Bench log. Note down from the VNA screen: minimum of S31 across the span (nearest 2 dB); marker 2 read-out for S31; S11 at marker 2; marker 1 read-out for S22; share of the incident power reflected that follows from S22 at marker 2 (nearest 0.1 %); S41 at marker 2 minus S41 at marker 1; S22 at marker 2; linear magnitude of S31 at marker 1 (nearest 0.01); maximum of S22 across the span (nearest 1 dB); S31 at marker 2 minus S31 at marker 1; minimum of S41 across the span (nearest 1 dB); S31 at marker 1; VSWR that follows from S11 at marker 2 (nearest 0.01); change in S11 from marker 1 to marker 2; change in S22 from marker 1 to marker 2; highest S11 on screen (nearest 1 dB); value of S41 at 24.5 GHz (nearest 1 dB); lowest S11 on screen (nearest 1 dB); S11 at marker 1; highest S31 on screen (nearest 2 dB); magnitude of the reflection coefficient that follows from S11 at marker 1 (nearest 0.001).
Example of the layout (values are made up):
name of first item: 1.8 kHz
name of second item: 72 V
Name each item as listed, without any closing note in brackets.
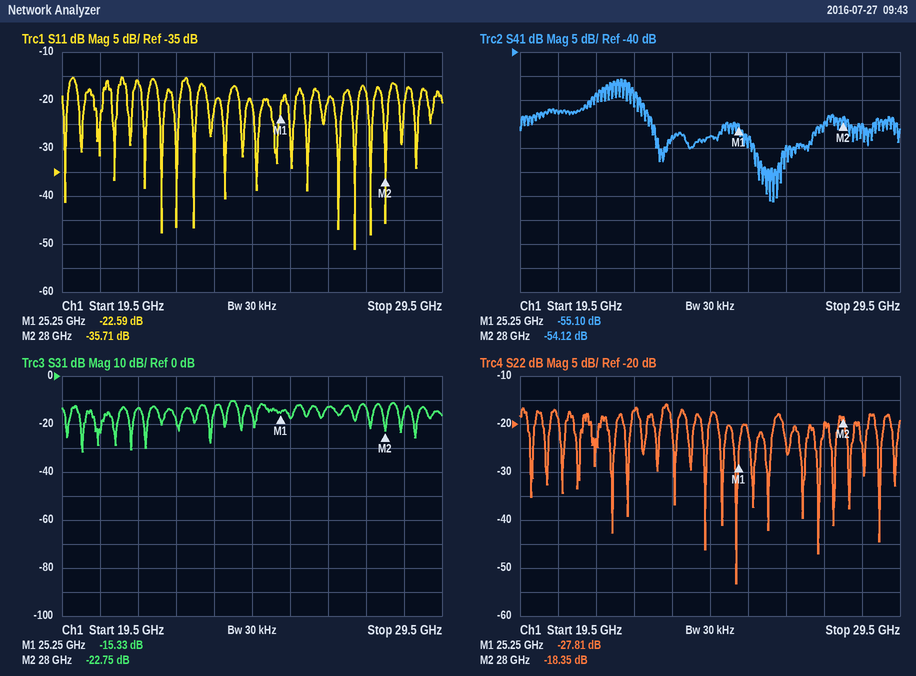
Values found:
minimum of S31 across the span: -32 dB
marker 2 read-out for S31: -22.75 dB
S11 at marker 2: -35.71 dB
marker 1 read-out for S22: -27.81 dB
share of the incident power reflected that follows from S22 at marker 2: 1.5 %
S41 at marker 2 minus S41 at marker 1: 0.98 dB
S22 at marker 2: -18.35 dB
linear magnitude of S31 at marker 1: 0.17
maximum of S22 across the span: -16 dB
S31 at marker 2 minus S31 at marker 1: -7.42 dB
minimum of S41 across the span: -71 dB
S31 at marker 1: -15.33 dB
VSWR that follows from S11 at marker 2: 1.03
change in S11 from marker 1 to marker 2: -13.12 dB
change in S22 from marker 1 to marker 2: 9.46 dB
highest S11 on screen: -15 dB
value of S41 at 24.5 GHz: -58 dB
lowest S11 on screen: -51 dB
S11 at marker 1: -22.59 dB
highest S31 on screen: -10 dB
magnitude of the reflection coefficient that follows from S11 at marker 1: 0.074
